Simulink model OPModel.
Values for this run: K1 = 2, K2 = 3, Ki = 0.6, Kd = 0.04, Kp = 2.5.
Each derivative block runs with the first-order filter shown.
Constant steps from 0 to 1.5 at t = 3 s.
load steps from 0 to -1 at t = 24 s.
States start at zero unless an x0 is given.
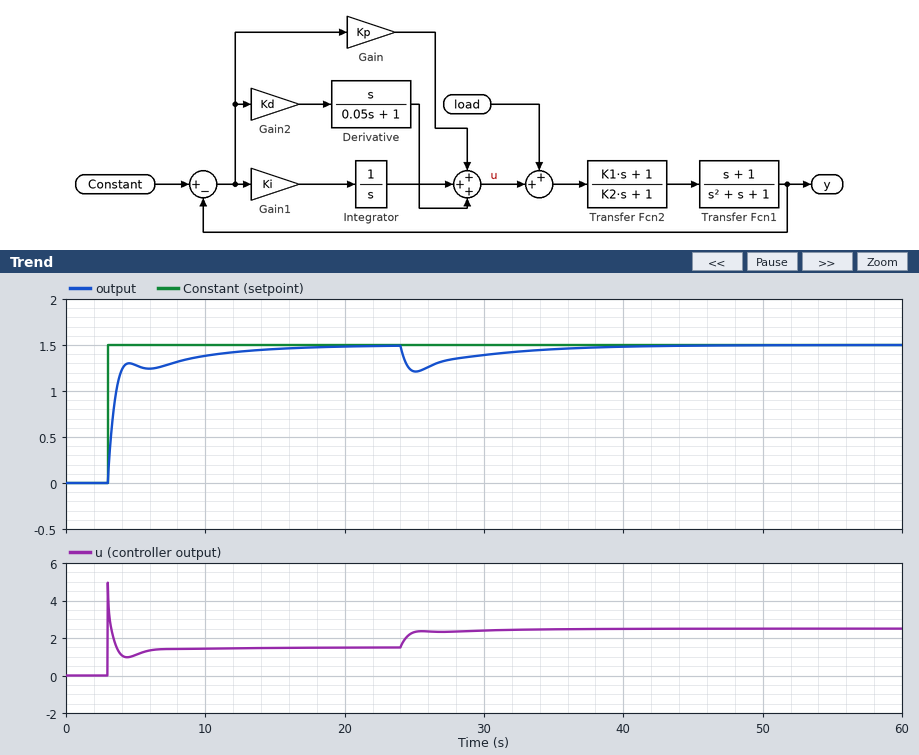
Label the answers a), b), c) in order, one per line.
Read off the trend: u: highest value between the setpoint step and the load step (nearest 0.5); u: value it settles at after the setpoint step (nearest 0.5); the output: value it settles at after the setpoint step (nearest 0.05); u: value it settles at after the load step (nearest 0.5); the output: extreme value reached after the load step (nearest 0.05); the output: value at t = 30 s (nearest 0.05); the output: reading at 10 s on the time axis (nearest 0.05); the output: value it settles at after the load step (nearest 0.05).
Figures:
a) 5.0
b) 1.5
c) 1.50
d) 2.5
e) 1.20
f) 1.40
g) 1.40
h) 1.50
